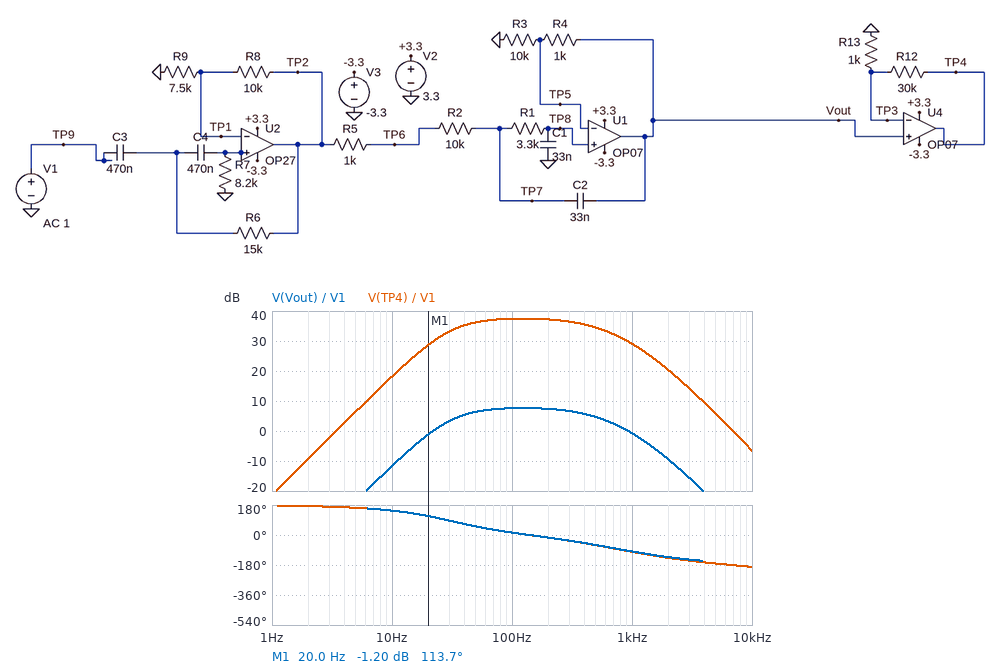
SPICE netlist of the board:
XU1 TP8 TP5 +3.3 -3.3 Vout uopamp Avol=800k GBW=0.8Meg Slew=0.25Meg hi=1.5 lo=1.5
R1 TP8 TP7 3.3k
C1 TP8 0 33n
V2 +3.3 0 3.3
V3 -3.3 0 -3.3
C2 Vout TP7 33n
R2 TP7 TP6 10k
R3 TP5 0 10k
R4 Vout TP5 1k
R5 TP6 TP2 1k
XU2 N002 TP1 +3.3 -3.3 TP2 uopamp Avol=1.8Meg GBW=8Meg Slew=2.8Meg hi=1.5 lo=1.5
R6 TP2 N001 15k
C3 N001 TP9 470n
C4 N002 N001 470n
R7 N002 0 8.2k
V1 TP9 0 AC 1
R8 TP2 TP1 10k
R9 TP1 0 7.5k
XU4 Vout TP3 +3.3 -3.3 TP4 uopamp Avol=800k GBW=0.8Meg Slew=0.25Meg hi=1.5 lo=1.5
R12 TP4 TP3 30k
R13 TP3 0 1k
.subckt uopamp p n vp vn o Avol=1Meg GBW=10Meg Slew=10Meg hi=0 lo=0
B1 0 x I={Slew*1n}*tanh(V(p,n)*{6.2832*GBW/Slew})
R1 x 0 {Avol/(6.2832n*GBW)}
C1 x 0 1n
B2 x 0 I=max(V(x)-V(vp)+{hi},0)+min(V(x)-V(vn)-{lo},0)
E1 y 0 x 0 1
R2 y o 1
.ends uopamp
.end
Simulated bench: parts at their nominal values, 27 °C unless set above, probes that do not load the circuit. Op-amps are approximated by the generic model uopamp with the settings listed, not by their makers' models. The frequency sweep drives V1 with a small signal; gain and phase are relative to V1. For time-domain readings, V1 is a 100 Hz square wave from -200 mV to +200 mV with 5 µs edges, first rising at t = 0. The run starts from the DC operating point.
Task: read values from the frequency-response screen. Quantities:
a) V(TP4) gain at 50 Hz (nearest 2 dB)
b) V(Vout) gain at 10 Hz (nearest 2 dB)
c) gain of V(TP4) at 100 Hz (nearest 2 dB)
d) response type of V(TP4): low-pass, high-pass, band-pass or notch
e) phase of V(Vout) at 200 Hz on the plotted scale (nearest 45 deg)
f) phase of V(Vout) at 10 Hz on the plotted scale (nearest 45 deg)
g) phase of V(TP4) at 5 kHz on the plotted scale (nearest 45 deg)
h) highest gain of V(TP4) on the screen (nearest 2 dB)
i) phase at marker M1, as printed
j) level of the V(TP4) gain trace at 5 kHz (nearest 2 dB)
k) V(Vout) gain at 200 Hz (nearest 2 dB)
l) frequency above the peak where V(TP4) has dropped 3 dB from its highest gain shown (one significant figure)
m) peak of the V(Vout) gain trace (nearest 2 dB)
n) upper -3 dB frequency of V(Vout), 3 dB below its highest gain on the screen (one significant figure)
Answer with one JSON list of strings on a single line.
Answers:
["36 dB", "-12 dB", "38 dB", "band-pass", "0 deg", "135 deg", "-180 deg", "38 dB", "113.7 deg", "6 dB", "8 dB", "500 Hz", "8 dB", "500 Hz"]
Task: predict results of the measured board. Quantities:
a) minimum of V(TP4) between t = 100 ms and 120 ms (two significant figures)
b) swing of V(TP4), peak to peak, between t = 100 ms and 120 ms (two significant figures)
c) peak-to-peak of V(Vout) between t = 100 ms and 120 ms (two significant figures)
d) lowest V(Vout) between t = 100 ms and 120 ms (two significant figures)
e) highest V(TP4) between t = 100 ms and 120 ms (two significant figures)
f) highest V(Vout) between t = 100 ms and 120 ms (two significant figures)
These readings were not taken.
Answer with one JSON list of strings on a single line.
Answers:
["-1.8 V", "3.6 V", "1.4 V", "-700 mV", "1.8 V", "700 mV"]
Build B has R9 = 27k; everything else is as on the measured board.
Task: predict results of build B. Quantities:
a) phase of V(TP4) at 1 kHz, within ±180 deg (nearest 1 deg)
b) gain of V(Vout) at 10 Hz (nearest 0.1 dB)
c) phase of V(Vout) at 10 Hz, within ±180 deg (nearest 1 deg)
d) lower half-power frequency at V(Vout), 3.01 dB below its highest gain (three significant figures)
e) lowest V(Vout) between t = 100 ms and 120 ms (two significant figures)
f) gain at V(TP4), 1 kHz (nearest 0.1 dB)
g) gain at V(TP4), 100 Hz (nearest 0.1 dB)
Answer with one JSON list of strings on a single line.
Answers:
["-100 deg", "-17.4 dB", "137 deg", "51.2 Hz", "-410 mV", "24.4 dB", "31.8 dB"]
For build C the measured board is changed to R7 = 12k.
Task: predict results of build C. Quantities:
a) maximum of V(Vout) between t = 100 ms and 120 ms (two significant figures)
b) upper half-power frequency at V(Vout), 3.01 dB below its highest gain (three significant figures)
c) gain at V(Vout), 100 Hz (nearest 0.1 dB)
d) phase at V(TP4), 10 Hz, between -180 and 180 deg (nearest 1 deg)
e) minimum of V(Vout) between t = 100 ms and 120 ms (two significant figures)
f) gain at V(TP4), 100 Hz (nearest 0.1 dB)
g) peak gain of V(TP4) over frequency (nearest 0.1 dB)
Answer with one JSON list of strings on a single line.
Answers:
["630 mV", "359 Hz", "8.2 dB", "152 deg", "-630 mV", "38.1 dB", "39.0 dB"]
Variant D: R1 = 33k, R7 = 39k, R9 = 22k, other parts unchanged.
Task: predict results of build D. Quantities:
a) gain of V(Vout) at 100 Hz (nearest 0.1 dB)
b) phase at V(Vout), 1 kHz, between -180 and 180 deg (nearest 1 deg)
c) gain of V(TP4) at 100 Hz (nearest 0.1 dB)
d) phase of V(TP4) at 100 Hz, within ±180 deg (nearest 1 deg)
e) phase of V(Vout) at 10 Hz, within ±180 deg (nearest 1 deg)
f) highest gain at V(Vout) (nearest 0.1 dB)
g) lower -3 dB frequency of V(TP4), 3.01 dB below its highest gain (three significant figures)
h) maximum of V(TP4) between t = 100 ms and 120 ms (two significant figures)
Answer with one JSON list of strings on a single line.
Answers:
["2.5 dB", "-148 deg", "32.3 dB", "-43 deg", "138 deg", "10.2 dB", "12.0 Hz", "1.8 V"]
